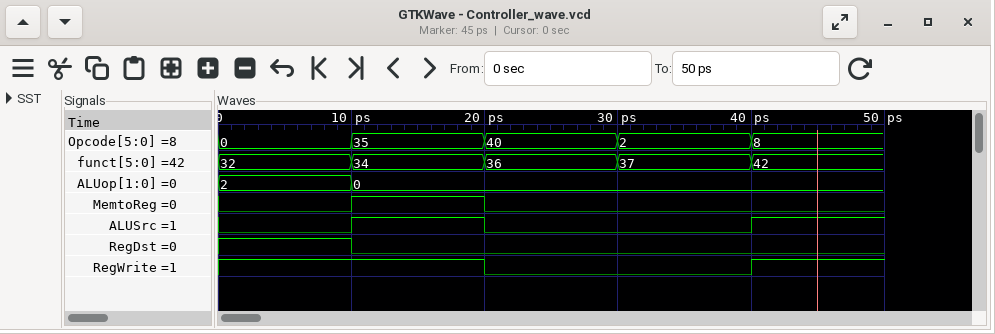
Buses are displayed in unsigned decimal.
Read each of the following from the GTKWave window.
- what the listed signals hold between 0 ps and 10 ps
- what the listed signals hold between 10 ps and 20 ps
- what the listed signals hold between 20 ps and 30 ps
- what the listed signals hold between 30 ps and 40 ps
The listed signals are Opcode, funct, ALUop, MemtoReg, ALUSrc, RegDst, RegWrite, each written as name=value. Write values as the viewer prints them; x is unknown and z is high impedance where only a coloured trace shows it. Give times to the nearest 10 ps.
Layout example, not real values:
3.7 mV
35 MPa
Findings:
Opcode=0, funct=32, ALUop=2, MemtoReg=0, ALUSrc=0, RegDst=1, RegWrite=1
Opcode=35, funct=34, ALUop=0, MemtoReg=1, ALUSrc=1, RegDst=0, RegWrite=1
Opcode=40, funct=36, ALUop=0, MemtoReg=0, ALUSrc=0, RegDst=0, RegWrite=0
Opcode=2, funct=37, ALUop=0, MemtoReg=0, ALUSrc=0, RegDst=0, RegWrite=0
